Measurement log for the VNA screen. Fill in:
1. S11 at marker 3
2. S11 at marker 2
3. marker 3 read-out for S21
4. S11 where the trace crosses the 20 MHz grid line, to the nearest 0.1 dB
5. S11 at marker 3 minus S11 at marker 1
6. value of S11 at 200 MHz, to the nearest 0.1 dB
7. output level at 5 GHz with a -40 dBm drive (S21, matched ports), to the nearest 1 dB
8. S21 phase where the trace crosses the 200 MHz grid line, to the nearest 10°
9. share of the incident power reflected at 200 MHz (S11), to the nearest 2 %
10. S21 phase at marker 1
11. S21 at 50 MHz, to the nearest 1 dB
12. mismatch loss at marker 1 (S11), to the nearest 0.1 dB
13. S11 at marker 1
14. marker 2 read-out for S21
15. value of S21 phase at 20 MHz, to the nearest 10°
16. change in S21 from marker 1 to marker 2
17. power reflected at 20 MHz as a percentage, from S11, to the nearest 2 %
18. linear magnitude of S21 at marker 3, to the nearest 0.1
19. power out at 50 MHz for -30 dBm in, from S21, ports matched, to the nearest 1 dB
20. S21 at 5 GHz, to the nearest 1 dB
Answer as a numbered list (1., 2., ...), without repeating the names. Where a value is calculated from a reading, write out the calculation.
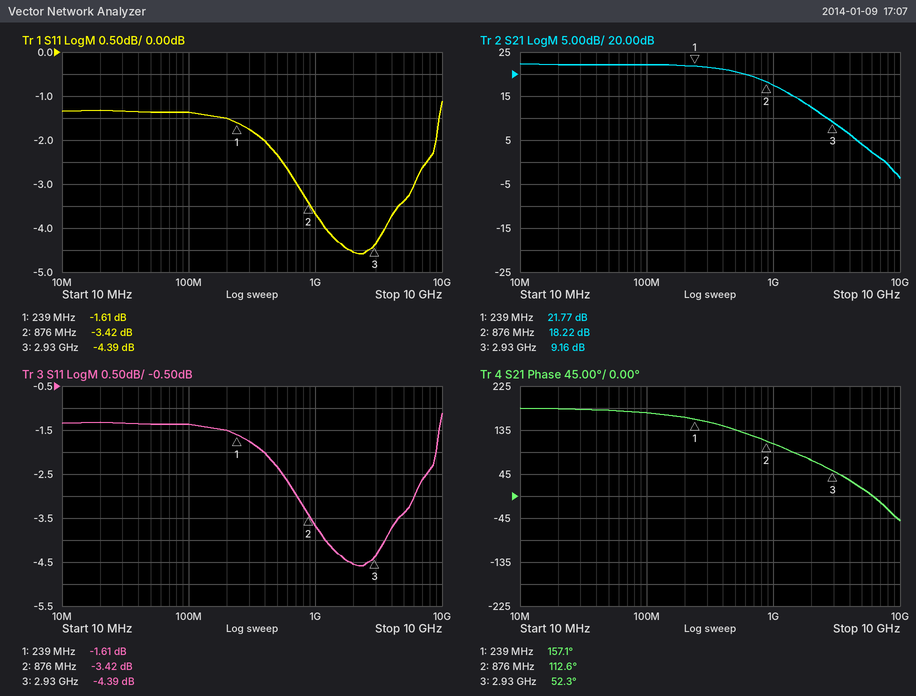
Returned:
1. -4.39 dB
2. -3.42 dB
3. 9.16 dB
4. -1.3 dB
5. -4.39 − (-1.61) = -2.78 dB
6. -1.5 dB
7. -40 dBm + (4 dB) = -36 dBm
8. 160°
9. 10^(-1.5/10) ≈ 70.8 %, so 70 % to the nearest 2 %
10. 157.1°
11. 22 dB
12. −10 log10(1 − 10^(-1.61/10)) ≈ 5.1 dB
13. -1.61 dB
14. 18.22 dB
15. 180°
16. 18.22 − (21.77) = -3.55 dB
17. 10^(-1.3/10) ≈ 74 %
18. 10^(9.16/20) ≈ 2.9
19. -30 dBm + (22 dB) = -8 dBm
20. 4 dB
